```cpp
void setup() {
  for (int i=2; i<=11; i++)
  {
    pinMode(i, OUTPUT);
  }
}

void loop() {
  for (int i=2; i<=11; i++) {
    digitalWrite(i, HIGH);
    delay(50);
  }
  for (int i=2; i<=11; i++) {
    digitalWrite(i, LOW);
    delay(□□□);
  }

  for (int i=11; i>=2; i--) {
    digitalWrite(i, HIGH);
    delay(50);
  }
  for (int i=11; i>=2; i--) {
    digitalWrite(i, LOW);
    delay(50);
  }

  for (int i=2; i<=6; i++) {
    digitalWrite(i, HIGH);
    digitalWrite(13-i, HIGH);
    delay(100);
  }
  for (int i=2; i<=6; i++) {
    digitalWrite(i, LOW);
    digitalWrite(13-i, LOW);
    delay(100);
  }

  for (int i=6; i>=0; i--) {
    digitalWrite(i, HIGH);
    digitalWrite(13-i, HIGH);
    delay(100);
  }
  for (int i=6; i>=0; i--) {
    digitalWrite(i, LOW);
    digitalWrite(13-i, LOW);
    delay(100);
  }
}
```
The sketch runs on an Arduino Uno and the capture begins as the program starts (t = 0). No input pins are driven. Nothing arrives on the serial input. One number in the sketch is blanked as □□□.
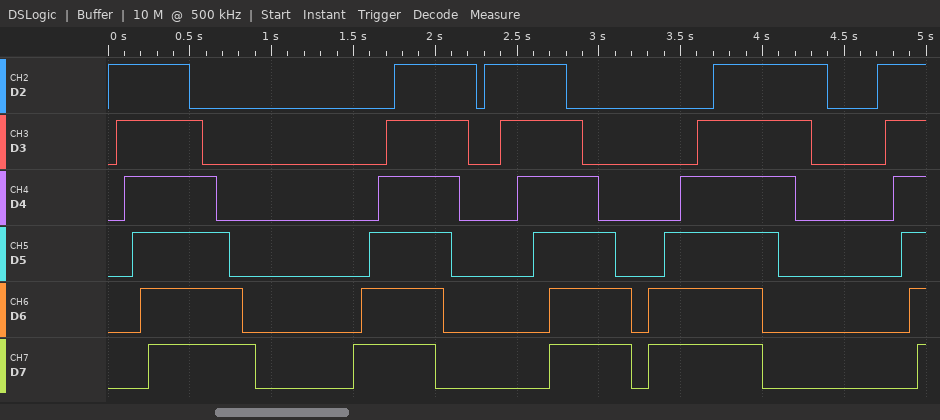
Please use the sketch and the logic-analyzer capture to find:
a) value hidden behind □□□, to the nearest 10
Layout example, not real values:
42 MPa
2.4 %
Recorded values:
80
